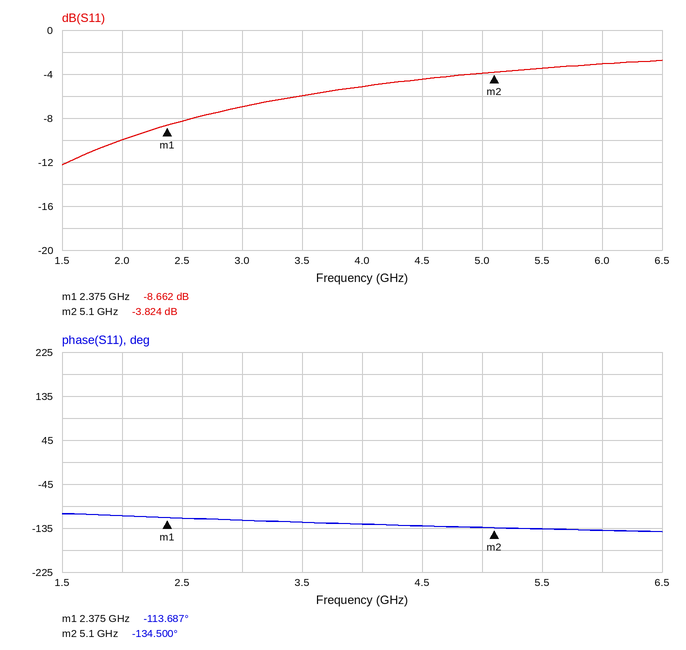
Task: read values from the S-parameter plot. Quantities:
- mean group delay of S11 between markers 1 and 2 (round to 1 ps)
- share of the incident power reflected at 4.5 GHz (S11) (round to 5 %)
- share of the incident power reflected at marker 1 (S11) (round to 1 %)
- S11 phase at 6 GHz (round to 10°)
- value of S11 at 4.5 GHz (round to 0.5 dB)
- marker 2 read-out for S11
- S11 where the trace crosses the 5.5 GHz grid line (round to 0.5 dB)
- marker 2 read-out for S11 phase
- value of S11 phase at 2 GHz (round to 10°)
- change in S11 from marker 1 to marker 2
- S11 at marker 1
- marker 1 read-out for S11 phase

21 ps
35 %
14 %
-140°
-4.5 dB
-3.824 dB
-3.5 dB
-134.500°
-110°
4.838 dB
-8.662 dB
-113.687°
